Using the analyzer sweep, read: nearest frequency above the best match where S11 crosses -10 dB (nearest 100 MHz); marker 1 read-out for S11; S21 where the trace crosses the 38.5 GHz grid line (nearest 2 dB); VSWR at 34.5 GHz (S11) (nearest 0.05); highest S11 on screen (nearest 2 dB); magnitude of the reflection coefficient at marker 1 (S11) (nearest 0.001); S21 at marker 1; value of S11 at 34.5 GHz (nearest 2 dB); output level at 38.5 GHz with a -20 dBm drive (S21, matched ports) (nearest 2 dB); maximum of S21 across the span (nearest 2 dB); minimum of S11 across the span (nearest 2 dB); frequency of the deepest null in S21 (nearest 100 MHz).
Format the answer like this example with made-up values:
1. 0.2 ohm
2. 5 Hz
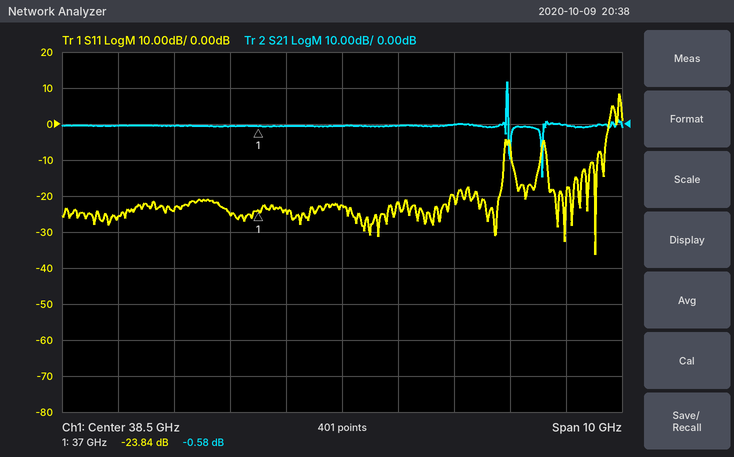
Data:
1. 43.1 GHz
2. -23.84 dB
3. 0 dB
4. 1.10
5. 8 dB
6. 0.064
7. -0.58 dB
8. -26 dB
9. -20 dBm
10. 12 dB
11. -36 dB
12. 42.1 GHz
